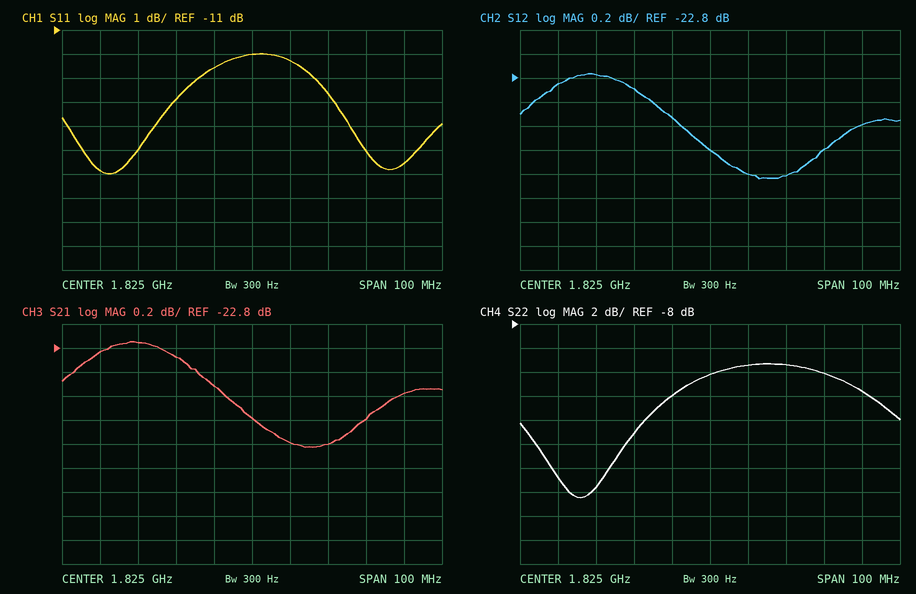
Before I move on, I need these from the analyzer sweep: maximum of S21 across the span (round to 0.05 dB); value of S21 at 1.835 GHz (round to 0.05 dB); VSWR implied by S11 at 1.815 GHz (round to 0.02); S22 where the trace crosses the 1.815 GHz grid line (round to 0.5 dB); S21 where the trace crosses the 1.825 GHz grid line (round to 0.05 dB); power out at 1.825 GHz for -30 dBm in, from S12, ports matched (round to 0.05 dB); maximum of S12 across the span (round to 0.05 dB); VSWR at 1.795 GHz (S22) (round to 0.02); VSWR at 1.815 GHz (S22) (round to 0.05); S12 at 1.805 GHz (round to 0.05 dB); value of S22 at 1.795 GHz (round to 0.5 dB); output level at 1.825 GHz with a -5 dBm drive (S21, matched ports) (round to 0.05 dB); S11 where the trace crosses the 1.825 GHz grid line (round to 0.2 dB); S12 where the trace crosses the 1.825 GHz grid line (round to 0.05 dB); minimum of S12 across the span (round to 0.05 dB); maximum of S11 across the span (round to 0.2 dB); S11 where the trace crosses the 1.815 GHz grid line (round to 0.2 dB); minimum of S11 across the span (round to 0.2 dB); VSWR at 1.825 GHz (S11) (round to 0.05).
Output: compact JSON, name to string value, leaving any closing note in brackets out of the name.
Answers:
{"maximum of S21 across the span": "-22.75 dB", "value of S21 at 1.835 GHz": "-23.60 dB", "VSWR implied by S11 at 1.815 GHz": "1.62", "S22 where the trace crosses the 1.815 GHz grid line": "-14.0 dB", "S21 where the trace crosses the 1.825 GHz grid line": "-23.40 dB", "power out at 1.825 GHz for -30 dBm in, from S12, ports matched": "-53.40 dBm", "maximum of S12 across the span": "-22.75 dB", "VSWR at 1.795 GHz (S22)": "1.18", "VSWR at 1.815 GHz (S22)": "1.50", "S12 at 1.805 GHz": "-22.90 dB", "value of S22 at 1.795 GHz": "-21.5 dB", "output level at 1.825 GHz with a -5 dBm drive (S21, matched ports)": "-28.40 dBm", "S11 where the trace crosses the 1.825 GHz grid line": "-12.0 dB", "S12 where the trace crosses the 1.825 GHz grid line": "-23.40 dB", "minimum of S12 across the span": "-23.65 dB", "maximum of S11 across the span": "-12.0 dB", "S11 where the trace crosses the 1.815 GHz grid line": "-12.6 dB", "minimum of S11 across the span": "-17.0 dB", "VSWR at 1.825 GHz (S11)": "1.65"}
